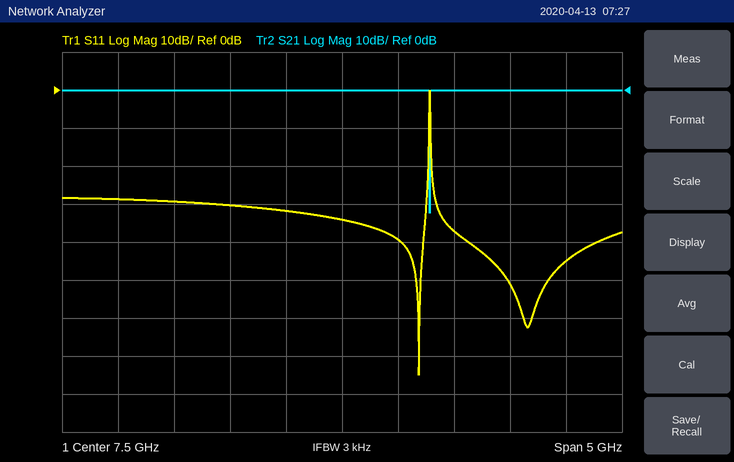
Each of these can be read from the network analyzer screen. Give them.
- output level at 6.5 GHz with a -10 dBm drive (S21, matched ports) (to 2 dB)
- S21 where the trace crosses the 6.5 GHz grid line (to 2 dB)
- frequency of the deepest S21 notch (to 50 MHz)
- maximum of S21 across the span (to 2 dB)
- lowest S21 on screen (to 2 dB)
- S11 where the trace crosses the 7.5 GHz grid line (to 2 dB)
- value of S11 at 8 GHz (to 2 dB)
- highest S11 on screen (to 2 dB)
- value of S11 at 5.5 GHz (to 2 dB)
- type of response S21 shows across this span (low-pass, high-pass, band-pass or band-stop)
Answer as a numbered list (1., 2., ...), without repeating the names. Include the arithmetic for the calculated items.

1. -10 dBm + (0 dB) = -10 dBm
2. 0 dB
3. 8.30 GHz
4. 0 dB
5. -32 dB
6. -34 dB
7. -40 dB
8. 0 dB
9. -28 dB
10. band-stop
